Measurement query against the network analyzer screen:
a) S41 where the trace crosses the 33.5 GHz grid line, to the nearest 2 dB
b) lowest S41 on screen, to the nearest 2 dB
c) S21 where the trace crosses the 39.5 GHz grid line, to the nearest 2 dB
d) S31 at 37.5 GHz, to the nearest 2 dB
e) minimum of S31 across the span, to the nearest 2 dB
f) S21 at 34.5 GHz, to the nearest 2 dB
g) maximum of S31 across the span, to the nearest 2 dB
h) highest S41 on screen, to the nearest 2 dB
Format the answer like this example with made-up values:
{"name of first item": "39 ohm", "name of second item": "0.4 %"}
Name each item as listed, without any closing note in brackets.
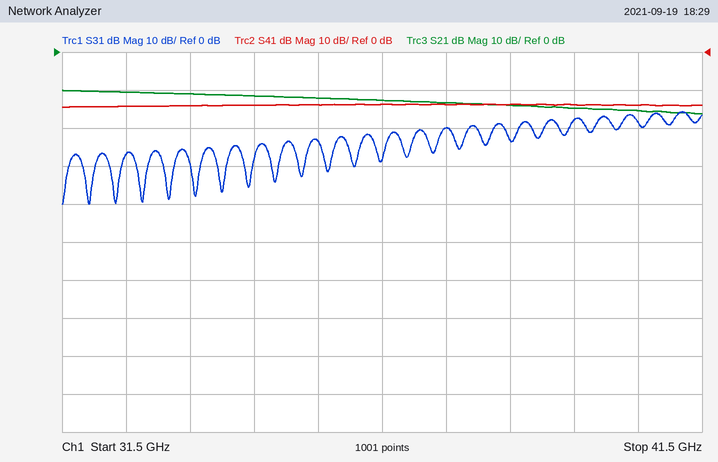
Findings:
{"S41 where the trace crosses the 33.5 GHz grid line, to the nearest 2 dB": "-14 dB", "lowest S41 on screen, to the nearest 2 dB": "-14 dB", "S21 where the trace crosses the 39.5 GHz grid line, to the nearest 2 dB": "-14 dB", "S31 at 37.5 GHz, to the nearest 2 dB": "-20 dB", "minimum of S31 across the span, to the nearest 2 dB": "-40 dB", "S21 at 34.5 GHz, to the nearest 2 dB": "-12 dB", "maximum of S31 across the span, to the nearest 2 dB": "-16 dB", "highest S41 on screen, to the nearest 2 dB": "-14 dB"}
